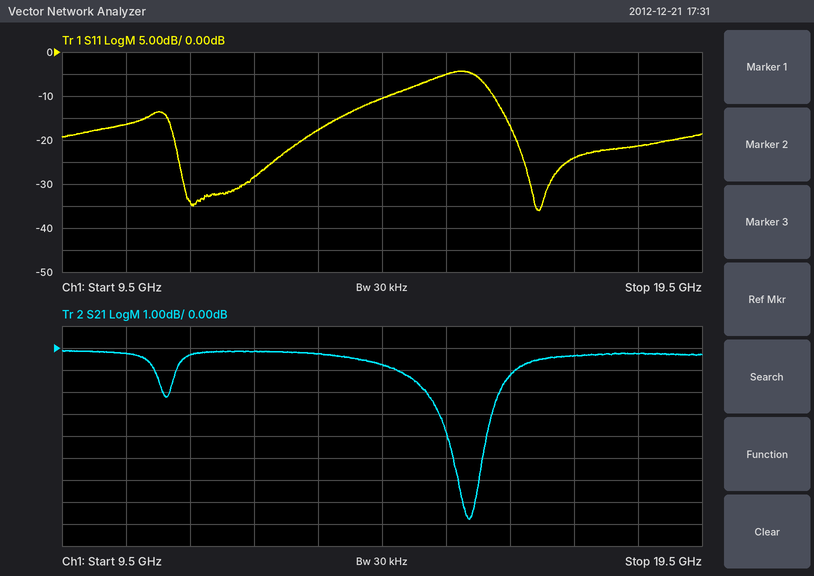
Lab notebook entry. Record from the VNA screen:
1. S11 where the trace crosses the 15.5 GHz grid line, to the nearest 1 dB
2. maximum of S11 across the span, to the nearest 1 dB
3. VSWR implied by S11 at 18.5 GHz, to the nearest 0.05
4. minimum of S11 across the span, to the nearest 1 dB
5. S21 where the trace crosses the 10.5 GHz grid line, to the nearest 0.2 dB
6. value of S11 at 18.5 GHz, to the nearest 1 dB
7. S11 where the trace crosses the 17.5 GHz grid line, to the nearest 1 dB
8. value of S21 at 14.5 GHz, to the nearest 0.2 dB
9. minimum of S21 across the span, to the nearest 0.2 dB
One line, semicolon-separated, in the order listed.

-5 dB; -4 dB; 1.20; -36 dB; -0.2 dB; -21 dB; -24 dB; -0.8 dB; -7.8 dB
